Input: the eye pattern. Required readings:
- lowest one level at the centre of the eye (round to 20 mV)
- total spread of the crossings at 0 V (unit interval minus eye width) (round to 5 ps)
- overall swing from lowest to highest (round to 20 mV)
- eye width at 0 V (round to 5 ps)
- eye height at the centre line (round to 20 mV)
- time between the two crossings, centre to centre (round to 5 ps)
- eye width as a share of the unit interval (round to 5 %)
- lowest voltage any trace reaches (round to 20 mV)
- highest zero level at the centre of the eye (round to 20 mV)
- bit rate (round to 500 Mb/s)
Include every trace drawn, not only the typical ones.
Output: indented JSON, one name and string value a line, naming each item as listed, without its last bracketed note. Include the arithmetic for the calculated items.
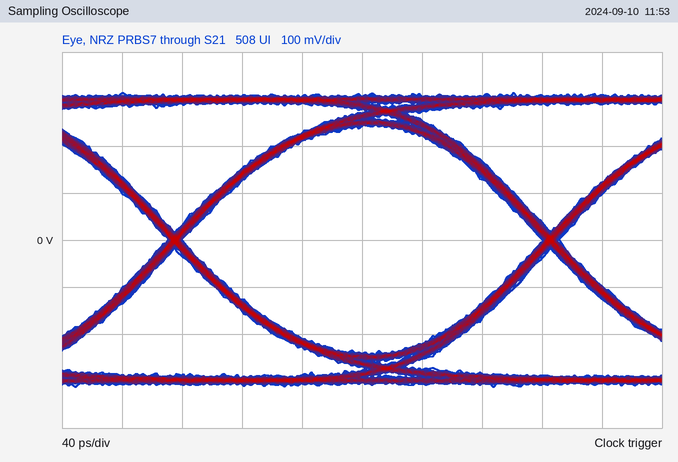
{
  "lowest one level at the centre of the eye": "240 mV",
  "total spread of the crossings at 0 V (unit interval minus eye width)": "10 ps",
  "overall swing from lowest to highest": "620 mV",
  "eye width at 0 V": "240 ps",
  "eye height at the centre line": "480 mV",
  "time between the two crossings, centre to centre": "250 ps",
  "eye width as a share of the unit interval": "240 ps / 250 ps ≈ 96.0 %, so 95 % to the nearest 5 %",
  "lowest voltage any trace reaches": "-320 mV",
  "highest zero level at the centre of the eye": "-240 mV",
  "bit rate": "4.0 Gb/s"
}
